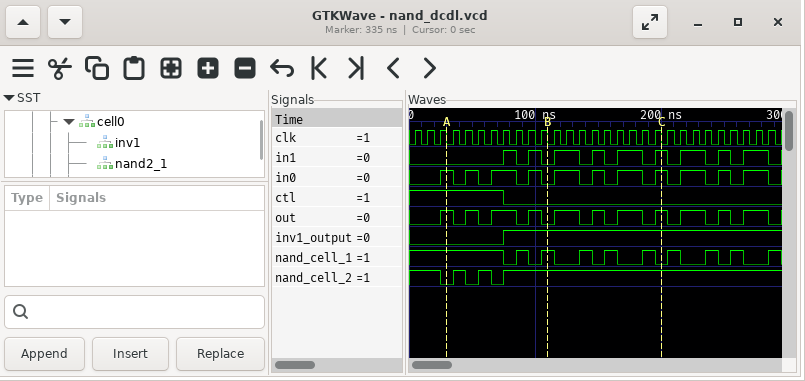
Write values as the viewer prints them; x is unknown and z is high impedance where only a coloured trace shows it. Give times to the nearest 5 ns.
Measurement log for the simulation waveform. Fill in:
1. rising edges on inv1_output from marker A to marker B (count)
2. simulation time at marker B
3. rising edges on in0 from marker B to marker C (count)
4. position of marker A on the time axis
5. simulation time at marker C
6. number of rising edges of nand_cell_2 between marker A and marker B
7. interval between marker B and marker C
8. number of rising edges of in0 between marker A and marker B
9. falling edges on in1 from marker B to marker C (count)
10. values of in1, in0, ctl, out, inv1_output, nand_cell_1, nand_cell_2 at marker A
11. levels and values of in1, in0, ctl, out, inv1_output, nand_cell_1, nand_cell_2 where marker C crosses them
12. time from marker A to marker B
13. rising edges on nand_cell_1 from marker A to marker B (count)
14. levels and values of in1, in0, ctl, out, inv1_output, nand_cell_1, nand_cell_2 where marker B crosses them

1
110 ns
4
30 ns
200 ns
3
90 ns
3
3
in1=0, in0=1, ctl=1, out=1, inv1_output=0, nand_cell_1=1, nand_cell_2=0
in1=1, in0=1, ctl=0, out=1, inv1_output=1, nand_cell_1=0, nand_cell_2=1
80 ns
2
in1=0, in0=0, ctl=0, out=0, inv1_output=1, nand_cell_1=1, nand_cell_2=1
